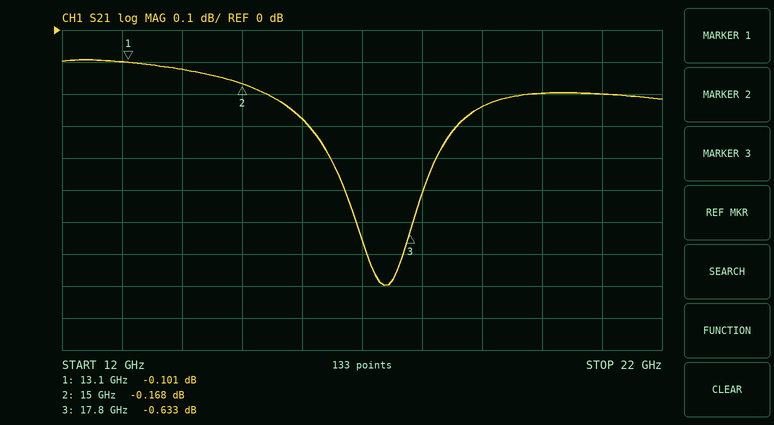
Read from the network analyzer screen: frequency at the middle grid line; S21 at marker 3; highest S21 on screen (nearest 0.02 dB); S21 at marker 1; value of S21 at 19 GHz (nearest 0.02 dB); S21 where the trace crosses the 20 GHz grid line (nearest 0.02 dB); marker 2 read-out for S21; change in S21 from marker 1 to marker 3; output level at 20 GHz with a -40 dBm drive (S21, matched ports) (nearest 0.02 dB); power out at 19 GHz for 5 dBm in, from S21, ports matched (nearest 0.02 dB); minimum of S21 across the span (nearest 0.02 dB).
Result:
17 GHz
-0.633 dB
-0.10 dB
-0.101 dB
-0.24 dB
-0.20 dB
-0.168 dB
-0.532 dB
-40.20 dBm
4.76 dBm
-0.80 dB
